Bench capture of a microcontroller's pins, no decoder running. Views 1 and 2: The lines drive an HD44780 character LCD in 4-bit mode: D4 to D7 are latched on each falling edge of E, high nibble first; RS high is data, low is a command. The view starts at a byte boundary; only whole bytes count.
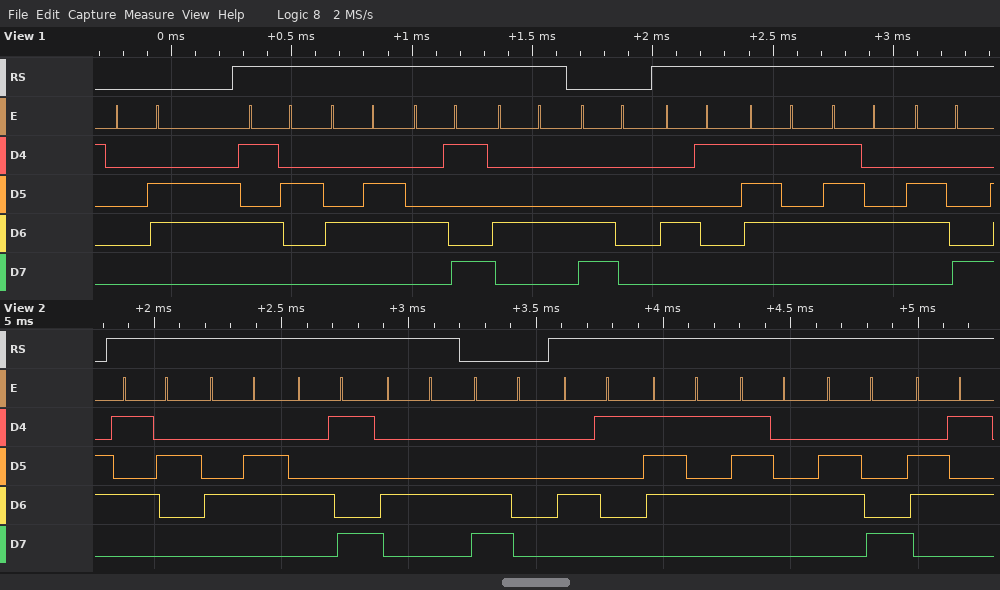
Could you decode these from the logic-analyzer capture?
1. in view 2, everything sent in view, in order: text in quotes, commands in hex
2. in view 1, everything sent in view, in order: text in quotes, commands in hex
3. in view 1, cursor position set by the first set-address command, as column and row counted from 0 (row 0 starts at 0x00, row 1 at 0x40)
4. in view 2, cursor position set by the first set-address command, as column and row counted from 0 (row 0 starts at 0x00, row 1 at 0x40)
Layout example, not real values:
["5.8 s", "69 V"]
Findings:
["\"RFID\" 0xC0 \"Authe\"", "0x06 \"RFID\" 0xC0 \"Auth\"", "column 0, row 1", "column 0, row 1"]
